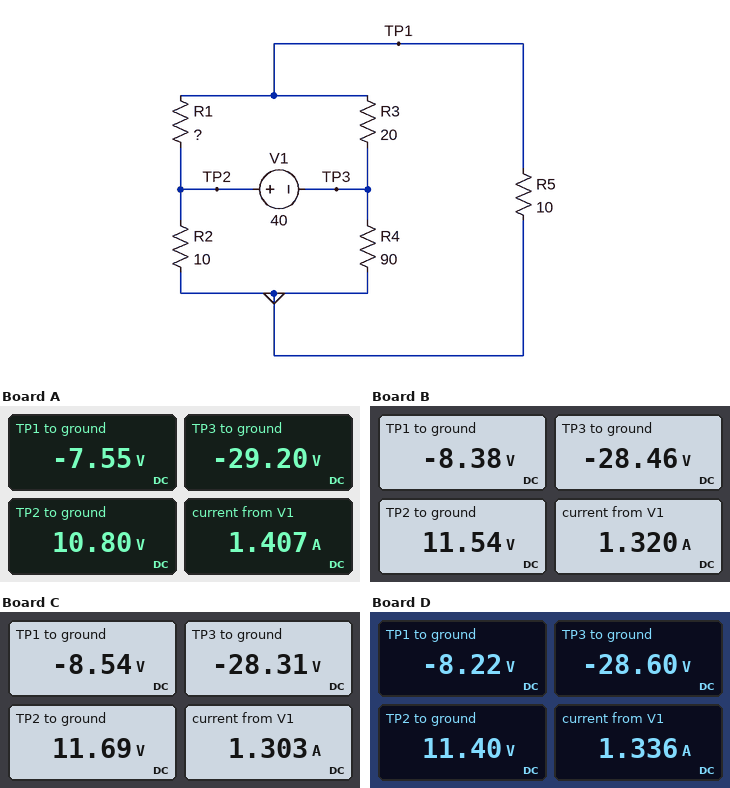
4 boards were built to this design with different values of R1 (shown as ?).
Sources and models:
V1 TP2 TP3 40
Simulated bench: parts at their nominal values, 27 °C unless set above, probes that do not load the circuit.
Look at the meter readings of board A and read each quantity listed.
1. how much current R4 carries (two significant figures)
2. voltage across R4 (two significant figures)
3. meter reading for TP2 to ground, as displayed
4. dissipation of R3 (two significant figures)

320 mA
29 V
10.80 V
23 W
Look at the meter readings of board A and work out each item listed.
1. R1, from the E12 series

56 Ω
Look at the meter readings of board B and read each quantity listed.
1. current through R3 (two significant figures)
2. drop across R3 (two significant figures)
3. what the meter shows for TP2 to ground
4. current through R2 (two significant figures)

1.0 A
20 V
11.54 V
1.2 A
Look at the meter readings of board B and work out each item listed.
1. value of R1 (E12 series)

120 Ω
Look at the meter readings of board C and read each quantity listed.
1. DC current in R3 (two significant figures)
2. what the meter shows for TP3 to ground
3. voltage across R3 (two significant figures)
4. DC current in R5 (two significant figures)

990 mA
-28.31 V
20 V
850 mA
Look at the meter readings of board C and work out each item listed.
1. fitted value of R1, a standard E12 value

150 Ω
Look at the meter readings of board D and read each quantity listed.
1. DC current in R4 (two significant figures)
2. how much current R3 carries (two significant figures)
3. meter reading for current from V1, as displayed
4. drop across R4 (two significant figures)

320 mA
1.0 A
1.336 A
29 V
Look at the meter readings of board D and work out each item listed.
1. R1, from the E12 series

100 Ω
